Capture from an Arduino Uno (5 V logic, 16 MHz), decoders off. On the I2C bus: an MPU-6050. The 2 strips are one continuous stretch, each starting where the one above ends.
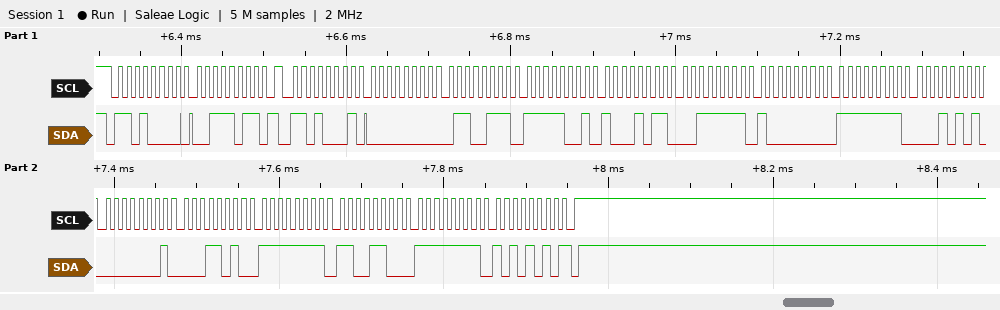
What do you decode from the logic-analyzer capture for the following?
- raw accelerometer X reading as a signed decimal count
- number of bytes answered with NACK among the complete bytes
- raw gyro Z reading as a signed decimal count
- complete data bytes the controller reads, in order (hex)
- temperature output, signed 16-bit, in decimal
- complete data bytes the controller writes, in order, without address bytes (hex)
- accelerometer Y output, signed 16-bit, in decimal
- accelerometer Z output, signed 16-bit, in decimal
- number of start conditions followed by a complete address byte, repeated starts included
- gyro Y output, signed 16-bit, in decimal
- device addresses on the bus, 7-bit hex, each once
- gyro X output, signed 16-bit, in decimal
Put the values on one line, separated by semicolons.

103; 1; -86; 00 67 F9 8B 3F 80 FF 15 01 1A FF CC FF AA; -235; 3B; -1653; 16256; 2; -52; 0x68; 282
